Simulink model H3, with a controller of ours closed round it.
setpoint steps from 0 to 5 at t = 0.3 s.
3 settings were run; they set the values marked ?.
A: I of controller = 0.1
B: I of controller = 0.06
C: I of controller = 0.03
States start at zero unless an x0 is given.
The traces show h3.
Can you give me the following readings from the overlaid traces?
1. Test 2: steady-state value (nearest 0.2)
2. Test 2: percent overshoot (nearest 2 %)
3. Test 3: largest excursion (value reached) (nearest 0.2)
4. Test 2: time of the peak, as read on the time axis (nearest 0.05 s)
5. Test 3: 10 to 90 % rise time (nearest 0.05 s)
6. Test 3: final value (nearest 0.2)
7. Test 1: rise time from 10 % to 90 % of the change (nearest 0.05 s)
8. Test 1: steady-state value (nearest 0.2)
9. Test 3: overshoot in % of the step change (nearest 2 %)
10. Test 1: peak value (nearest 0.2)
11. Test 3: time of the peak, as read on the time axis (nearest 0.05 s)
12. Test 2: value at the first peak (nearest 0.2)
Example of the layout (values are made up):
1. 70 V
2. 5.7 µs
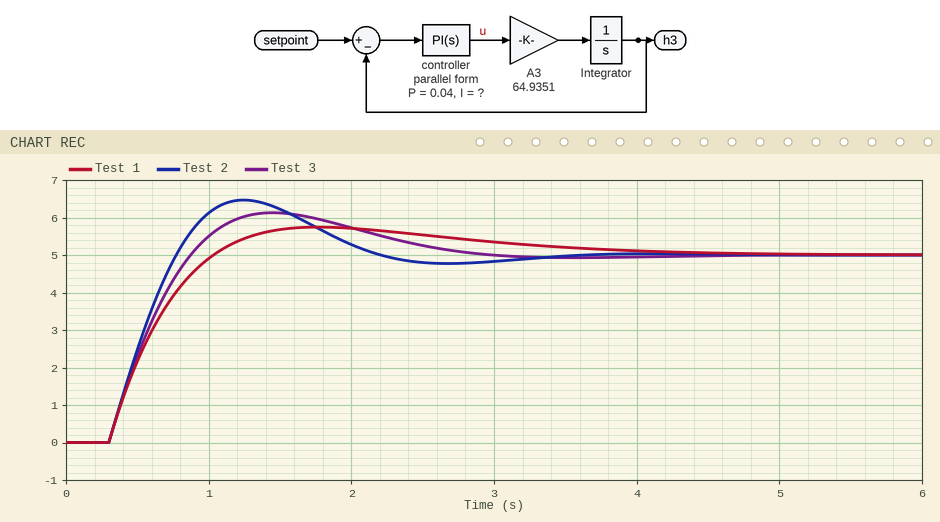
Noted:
1. 5.0
2. 30 %
3. 6.2
4. 1.25 s
5. 0.45 s
6. 5.0
7. 0.55 s
8. 5.0
9. 22 %
10. 5.8
11. 1.45 s
12. 6.4
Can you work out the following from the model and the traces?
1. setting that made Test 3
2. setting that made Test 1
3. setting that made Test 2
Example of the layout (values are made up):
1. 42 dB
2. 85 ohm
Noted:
1. B
2. C
3. A
